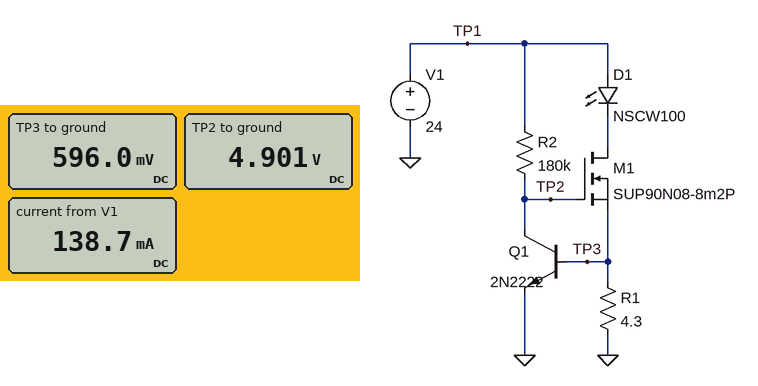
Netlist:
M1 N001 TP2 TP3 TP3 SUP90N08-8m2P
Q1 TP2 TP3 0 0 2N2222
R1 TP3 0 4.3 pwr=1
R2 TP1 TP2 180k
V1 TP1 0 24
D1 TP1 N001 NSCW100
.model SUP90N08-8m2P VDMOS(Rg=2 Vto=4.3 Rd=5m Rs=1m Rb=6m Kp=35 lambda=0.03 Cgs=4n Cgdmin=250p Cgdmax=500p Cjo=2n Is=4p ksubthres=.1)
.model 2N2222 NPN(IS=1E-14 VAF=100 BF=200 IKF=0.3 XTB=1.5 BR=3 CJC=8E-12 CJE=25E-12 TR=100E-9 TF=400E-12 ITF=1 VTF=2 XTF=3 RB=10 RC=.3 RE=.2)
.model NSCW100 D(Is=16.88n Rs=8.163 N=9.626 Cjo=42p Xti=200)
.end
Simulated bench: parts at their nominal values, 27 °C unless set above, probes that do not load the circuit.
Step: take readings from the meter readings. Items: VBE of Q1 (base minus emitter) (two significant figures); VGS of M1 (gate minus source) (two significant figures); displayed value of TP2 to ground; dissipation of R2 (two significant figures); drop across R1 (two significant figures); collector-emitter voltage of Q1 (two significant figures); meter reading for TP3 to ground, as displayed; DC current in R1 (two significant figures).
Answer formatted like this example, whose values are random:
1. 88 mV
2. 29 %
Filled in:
1. 600 mV
2. 4.3 V
3. 4.901 V
4. 2.0 mW
5. 600 mV
6. 4.9 V
7. 596.0 mV
8. 140 mA
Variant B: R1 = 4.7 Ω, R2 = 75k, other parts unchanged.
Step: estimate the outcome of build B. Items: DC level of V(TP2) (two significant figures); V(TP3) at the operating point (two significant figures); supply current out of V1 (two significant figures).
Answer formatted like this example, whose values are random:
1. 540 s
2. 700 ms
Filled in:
1. 4.9 V
2. 620 mV
3. 130 mA
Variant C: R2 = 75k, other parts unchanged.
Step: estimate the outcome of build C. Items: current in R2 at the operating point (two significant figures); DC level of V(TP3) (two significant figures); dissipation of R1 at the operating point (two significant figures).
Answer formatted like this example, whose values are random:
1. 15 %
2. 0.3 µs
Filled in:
1. 250 µA
2. 620 mV
3. 89 mW
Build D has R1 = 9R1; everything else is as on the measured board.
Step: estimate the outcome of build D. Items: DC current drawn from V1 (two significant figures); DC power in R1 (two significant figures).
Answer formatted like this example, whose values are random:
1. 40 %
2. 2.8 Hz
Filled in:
1. 66 mA
2. 39 mW
